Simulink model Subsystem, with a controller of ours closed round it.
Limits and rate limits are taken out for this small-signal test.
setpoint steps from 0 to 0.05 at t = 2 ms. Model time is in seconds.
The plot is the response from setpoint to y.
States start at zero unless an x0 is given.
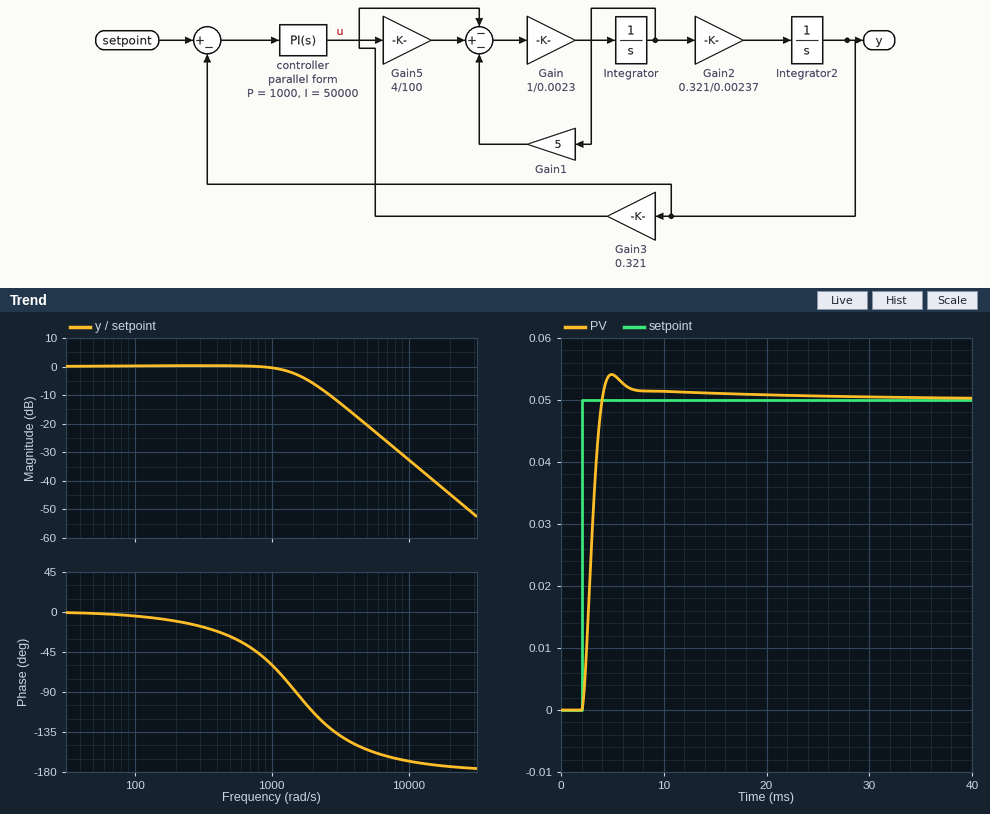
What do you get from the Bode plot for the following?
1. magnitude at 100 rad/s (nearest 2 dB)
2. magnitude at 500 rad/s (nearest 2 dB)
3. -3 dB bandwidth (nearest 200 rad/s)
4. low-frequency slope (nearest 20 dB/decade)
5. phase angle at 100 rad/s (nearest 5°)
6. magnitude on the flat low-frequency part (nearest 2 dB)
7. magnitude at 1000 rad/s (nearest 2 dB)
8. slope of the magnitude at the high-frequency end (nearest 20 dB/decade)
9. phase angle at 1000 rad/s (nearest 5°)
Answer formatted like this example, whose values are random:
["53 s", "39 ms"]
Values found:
["0 dB", "0 dB", "1600 rad/s", "0 dB/decade", "-5°", "0 dB", "0 dB", "-40 dB/decade", "-60°"]
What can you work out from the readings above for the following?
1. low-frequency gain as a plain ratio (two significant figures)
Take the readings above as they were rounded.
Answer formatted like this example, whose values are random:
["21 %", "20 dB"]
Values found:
["1.0"]
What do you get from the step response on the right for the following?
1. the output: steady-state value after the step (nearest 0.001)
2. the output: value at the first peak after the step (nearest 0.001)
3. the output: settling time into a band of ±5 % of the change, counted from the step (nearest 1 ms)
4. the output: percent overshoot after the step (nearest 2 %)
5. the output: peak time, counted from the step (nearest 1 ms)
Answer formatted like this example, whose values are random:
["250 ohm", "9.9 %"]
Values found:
["0.050", "0.054", "4 ms", "8 %", "3 ms"]
